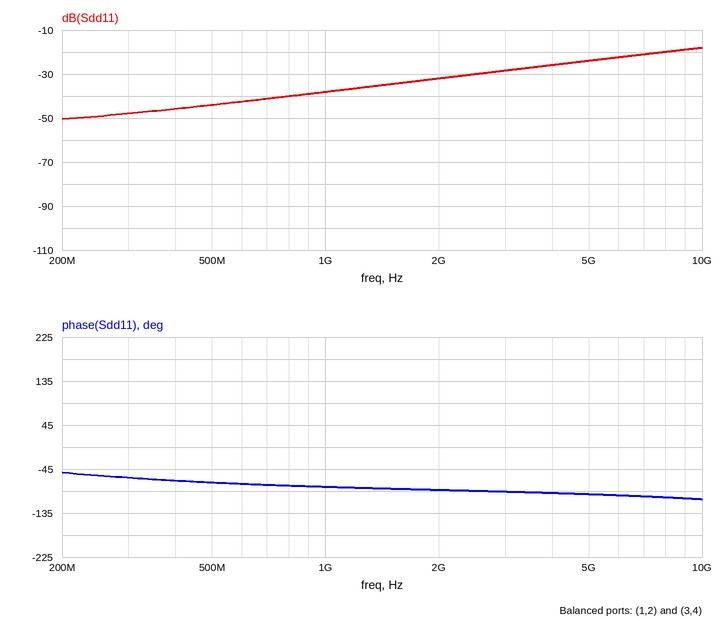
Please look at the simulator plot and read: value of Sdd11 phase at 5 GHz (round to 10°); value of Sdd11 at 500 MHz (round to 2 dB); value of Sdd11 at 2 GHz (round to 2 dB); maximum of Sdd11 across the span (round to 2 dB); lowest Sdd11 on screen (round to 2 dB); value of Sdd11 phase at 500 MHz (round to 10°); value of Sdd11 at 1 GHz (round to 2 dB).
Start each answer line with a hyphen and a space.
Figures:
- -100°
- -44 dB
- -32 dB
- -18 dB
- -50 dB
- -70°
- -38 dB
